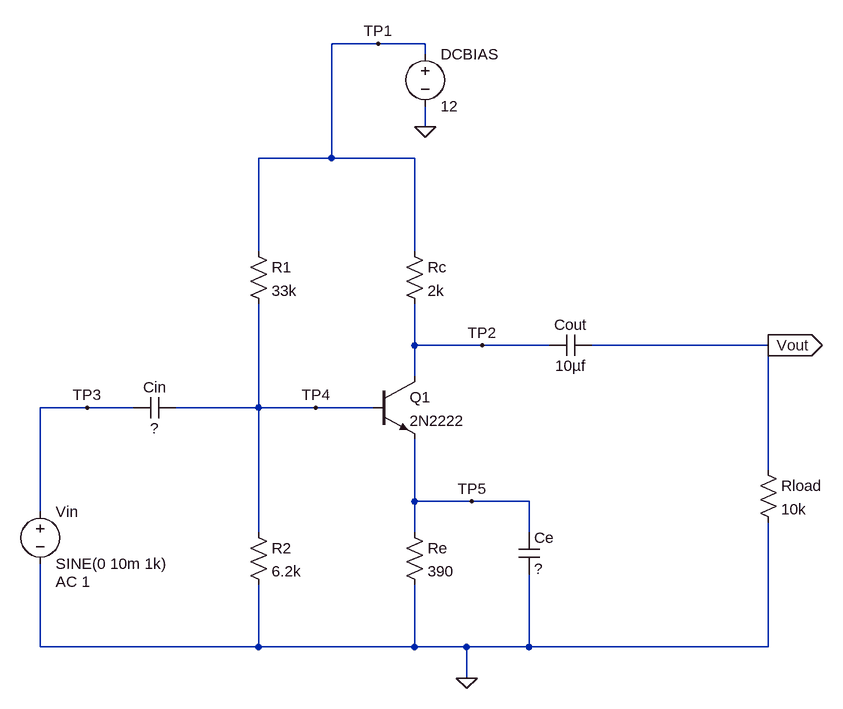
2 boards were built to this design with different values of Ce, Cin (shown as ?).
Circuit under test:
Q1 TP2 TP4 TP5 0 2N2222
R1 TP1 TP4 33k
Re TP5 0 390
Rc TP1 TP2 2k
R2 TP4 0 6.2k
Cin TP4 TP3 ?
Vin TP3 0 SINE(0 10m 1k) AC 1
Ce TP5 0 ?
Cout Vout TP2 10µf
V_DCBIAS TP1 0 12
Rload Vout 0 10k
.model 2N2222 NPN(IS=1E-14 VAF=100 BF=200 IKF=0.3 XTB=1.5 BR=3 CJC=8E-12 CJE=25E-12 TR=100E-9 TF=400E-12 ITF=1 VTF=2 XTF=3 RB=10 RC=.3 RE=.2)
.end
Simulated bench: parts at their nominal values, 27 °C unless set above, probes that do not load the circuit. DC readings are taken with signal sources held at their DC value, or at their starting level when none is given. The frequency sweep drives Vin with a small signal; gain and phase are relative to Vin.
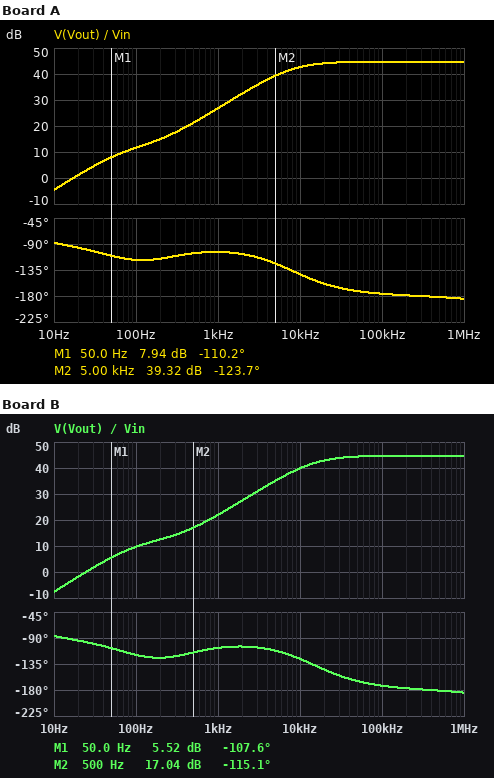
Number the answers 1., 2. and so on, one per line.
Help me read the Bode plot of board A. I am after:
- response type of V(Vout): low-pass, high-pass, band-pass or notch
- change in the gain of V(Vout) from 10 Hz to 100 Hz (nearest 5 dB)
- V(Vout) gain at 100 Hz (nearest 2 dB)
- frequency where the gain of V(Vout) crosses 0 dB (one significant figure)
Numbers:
1. high-pass
2. 15 dB
3. 12 dB
4. 20 Hz
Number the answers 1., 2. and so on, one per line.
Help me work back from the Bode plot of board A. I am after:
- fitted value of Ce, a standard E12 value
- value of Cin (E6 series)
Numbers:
1. 2.2 µF
2. 470 nF
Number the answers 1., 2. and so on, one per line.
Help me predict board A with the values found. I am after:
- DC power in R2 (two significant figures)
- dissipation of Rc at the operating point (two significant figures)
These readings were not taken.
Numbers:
1. 540 µW
2. 17 mW
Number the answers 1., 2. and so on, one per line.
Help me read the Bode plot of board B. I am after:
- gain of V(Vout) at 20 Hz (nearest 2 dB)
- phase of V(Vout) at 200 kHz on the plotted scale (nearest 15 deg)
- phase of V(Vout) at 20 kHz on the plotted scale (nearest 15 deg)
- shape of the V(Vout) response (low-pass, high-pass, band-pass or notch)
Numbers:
1. -2 dB
2. -180 deg
3. -150 deg
4. high-pass
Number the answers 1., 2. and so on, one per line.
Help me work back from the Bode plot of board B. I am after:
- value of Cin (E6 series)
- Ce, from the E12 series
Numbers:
1. 330 nF
2. 1.2 µF
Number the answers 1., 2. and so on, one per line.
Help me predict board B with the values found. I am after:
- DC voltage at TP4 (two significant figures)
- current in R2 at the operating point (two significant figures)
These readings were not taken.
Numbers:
1. 1.8 V
2. 290 µA
